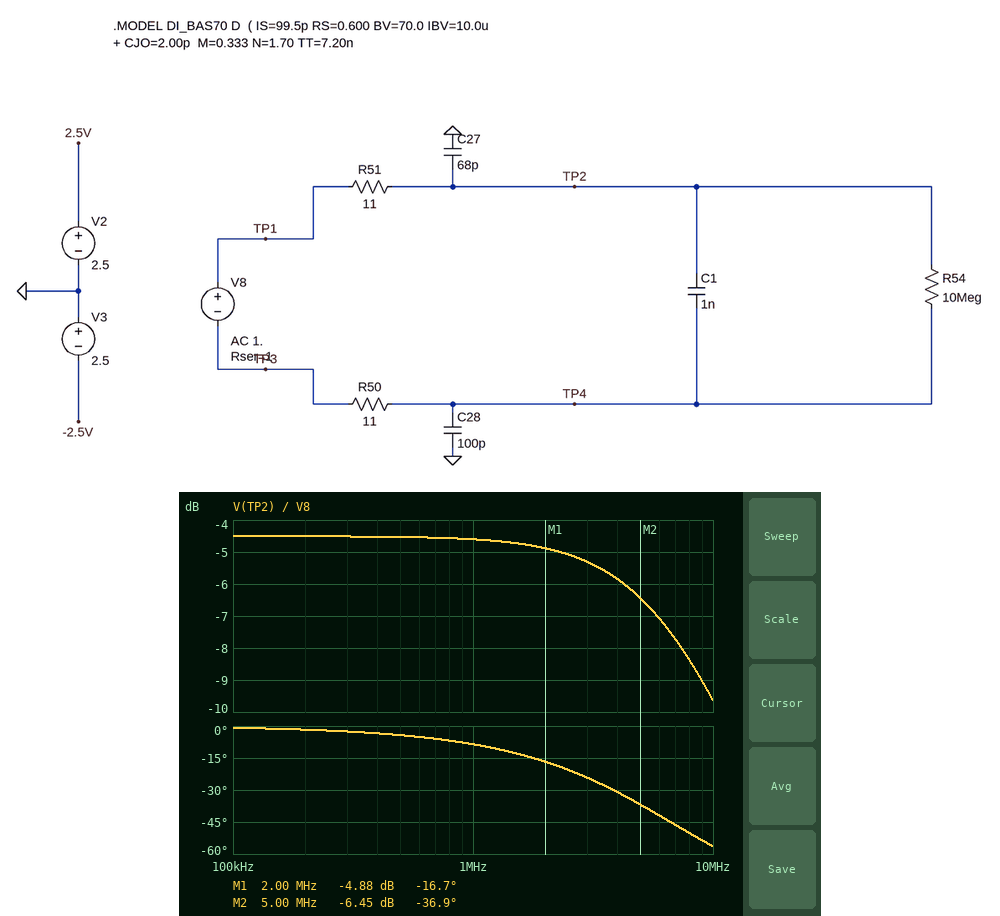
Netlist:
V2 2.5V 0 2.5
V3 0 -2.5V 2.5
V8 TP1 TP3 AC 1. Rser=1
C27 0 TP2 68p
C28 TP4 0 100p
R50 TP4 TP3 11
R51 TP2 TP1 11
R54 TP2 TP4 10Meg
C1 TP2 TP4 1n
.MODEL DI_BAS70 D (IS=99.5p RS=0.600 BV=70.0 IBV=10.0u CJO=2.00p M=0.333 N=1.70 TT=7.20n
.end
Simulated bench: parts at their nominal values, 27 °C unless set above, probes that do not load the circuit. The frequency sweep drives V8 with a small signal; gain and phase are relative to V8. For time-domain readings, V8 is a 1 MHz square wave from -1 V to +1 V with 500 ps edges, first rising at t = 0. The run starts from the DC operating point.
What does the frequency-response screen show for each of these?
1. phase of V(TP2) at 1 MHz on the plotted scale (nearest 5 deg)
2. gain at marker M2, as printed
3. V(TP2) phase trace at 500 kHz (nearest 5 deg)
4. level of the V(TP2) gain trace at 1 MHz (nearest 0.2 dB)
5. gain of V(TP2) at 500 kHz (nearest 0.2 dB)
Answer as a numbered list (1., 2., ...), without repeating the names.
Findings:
1. -10 deg
2. -6.45 dB
3. -5 deg
4. -4.6 dB
5. -4.6 dB
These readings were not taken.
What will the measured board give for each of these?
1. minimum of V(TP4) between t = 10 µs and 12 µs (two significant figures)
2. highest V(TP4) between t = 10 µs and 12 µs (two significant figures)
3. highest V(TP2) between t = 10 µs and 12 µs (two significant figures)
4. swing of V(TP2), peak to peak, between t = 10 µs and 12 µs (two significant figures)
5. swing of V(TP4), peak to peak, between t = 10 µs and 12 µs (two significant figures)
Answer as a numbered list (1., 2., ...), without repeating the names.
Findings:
1. 190 mV
2. 1.0 V
3. 1.2 V
4. 1.2 V
5. 810 mV
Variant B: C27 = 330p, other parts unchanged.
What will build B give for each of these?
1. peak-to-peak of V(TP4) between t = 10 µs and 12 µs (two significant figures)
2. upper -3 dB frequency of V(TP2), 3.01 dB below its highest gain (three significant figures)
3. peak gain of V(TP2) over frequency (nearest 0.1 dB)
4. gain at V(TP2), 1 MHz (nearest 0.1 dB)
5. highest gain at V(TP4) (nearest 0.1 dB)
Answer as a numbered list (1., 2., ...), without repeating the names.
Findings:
1. 1.5 V
2. 6.43 MHz
3. -12.7 dB
4. -12.8 dB
5. -2.3 dB
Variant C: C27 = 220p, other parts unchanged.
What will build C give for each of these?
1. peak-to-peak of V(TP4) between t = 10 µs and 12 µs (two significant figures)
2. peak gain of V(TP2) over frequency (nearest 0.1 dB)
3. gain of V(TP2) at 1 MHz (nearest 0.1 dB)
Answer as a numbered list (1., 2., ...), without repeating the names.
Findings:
1. 1.4 V
2. -10.1 dB
3. -10.2 dB
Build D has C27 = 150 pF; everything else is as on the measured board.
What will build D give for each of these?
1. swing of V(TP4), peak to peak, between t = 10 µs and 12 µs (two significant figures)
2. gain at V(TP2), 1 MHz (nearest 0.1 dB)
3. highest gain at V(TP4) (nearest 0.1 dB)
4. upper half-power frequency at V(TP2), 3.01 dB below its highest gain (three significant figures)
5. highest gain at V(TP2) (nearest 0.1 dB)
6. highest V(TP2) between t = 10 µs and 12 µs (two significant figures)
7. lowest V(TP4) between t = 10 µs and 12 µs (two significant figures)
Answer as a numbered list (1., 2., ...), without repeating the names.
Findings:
1. 1.2 V
2. -8.1 dB
3. -4.4 dB
4. 6.53 MHz
5. -8.0 dB
6. 800 mV
7. -200 mV
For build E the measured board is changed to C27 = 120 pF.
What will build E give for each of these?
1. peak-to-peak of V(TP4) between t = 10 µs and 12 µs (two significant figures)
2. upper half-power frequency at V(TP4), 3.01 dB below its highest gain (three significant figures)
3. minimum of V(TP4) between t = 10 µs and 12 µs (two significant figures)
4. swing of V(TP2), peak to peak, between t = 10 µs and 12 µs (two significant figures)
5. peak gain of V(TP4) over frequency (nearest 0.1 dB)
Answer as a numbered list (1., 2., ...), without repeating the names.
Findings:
1. 1.1 V
2. 6.56 MHz
3. -91 mV
4. 910 mV
5. -5.3 dB
